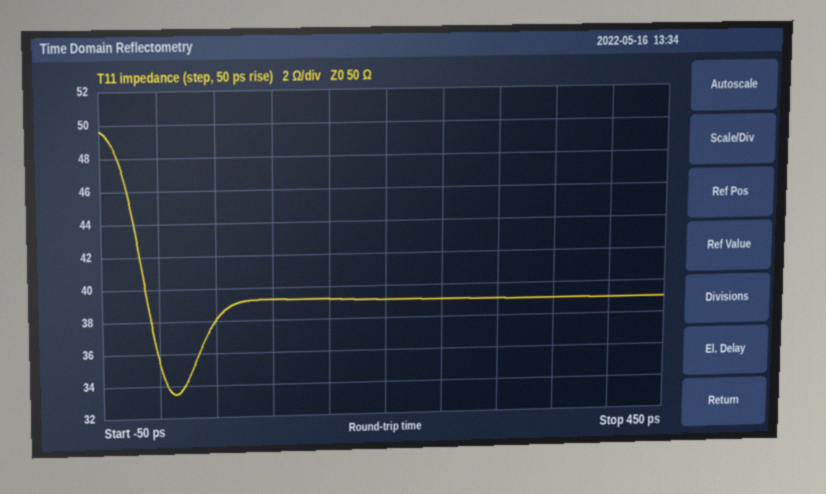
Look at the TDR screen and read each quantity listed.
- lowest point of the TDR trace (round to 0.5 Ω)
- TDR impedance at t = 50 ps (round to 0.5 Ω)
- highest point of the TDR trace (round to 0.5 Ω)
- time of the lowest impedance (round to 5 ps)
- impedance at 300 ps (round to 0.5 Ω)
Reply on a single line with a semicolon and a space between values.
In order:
33.5 Ω; 38.0 Ω; 49.5 Ω; 15 ps; 39.0 Ω
